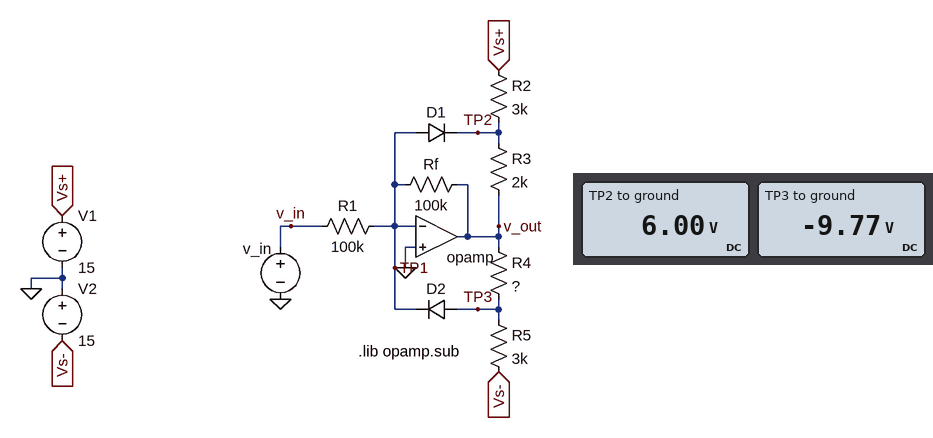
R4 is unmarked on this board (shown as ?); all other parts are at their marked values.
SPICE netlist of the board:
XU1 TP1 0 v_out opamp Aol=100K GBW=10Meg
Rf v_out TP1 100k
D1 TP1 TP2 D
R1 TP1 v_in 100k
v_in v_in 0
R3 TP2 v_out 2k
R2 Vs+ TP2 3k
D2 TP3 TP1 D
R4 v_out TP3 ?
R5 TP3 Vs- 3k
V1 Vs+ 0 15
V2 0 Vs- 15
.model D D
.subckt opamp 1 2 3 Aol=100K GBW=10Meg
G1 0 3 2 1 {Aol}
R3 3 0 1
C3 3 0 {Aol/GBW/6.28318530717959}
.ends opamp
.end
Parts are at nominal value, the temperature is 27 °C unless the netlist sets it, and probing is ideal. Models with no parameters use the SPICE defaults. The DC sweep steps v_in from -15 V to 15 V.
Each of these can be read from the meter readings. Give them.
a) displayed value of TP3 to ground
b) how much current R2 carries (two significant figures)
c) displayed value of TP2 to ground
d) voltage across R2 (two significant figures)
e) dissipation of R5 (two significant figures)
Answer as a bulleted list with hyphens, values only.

- -9.77 V
- 3.0 mA
- 6.00 V
- 9.0 V
- 9.1 mW
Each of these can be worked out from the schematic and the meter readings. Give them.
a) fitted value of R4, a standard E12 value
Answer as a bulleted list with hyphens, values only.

- 5.6 kΩ
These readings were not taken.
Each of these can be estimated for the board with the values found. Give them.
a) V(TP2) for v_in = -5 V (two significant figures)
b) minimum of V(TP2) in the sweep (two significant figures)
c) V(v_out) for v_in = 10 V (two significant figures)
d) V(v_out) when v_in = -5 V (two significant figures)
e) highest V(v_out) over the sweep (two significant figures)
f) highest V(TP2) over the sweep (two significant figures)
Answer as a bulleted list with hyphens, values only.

- 9.0 V
- -570 mV
- -10 V
- 5.0 V
- 15 V
- 15 V
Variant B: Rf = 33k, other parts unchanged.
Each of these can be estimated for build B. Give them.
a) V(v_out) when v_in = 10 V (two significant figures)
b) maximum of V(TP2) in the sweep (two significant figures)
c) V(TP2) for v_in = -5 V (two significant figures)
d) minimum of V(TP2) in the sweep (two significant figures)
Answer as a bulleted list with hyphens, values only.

- -3.3 V
- 9.0 V
- 7.0 V
- 3.0 V
